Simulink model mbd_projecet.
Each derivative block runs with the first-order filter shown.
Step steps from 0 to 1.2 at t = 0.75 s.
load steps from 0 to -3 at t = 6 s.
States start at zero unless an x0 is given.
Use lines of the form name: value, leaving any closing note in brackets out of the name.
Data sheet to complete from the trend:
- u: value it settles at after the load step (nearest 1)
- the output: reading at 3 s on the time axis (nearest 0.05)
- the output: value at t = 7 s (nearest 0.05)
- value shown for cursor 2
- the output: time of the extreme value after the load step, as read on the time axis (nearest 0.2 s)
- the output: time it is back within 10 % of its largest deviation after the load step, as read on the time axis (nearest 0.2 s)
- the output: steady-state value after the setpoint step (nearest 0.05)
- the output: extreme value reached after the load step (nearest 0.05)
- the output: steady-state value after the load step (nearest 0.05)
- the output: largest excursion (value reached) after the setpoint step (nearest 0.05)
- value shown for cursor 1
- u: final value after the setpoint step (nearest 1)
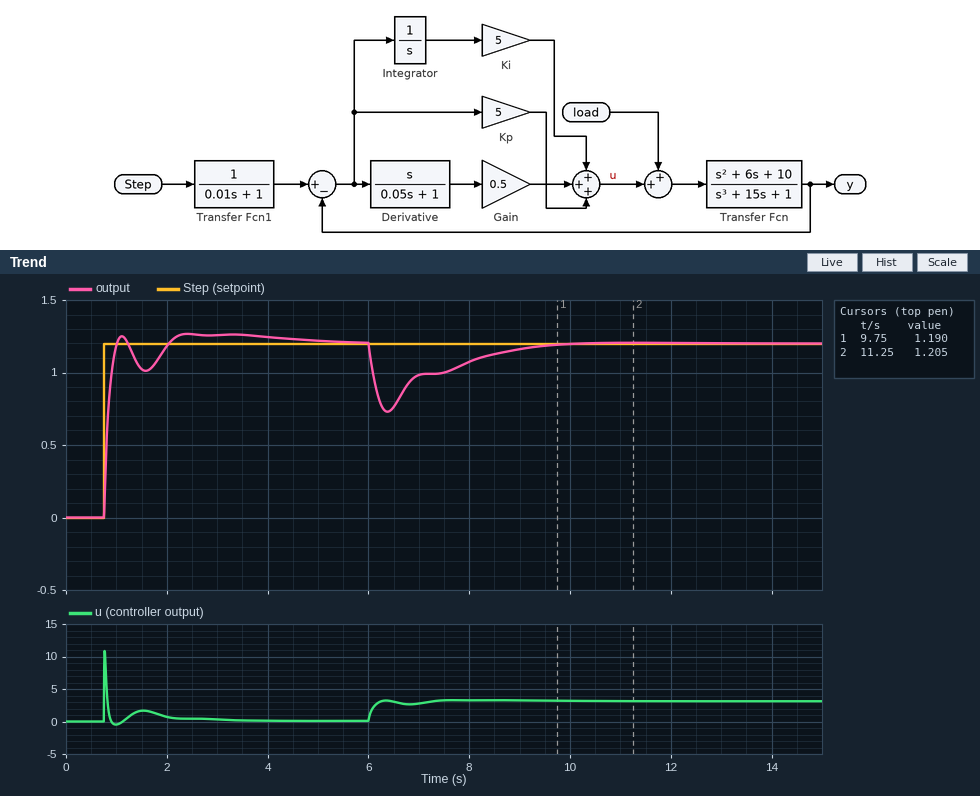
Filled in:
u: value it settles at after the load step: 3
the output: reading at 3 s on the time axis: 1.25
the output: value at t = 7 s: 1.00
value shown for cursor 2: 1.205
the output: time of the extreme value after the load step, as read on the time axis: 6.4 s
the output: time it is back within 10 % of its largest deviation after the load step, as read on the time axis: 8.8 s
the output: steady-state value after the setpoint step: 1.20
the output: extreme value reached after the load step: 0.75
the output: steady-state value after the load step: 1.20
the output: largest excursion (value reached) after the setpoint step: 1.25
value shown for cursor 1: 1.190
u: final value after the setpoint step: 0
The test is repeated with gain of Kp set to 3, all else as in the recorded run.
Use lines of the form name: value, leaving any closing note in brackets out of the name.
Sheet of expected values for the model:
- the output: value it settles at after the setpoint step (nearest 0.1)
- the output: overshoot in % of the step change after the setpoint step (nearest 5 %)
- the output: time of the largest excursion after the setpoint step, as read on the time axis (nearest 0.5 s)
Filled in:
the output: value it settles at after the setpoint step: 1.2
the output: overshoot in % of the step change after the setpoint step: 10 %
the output: time of the largest excursion after the setpoint step, as read on the time axis: 2.5 s
